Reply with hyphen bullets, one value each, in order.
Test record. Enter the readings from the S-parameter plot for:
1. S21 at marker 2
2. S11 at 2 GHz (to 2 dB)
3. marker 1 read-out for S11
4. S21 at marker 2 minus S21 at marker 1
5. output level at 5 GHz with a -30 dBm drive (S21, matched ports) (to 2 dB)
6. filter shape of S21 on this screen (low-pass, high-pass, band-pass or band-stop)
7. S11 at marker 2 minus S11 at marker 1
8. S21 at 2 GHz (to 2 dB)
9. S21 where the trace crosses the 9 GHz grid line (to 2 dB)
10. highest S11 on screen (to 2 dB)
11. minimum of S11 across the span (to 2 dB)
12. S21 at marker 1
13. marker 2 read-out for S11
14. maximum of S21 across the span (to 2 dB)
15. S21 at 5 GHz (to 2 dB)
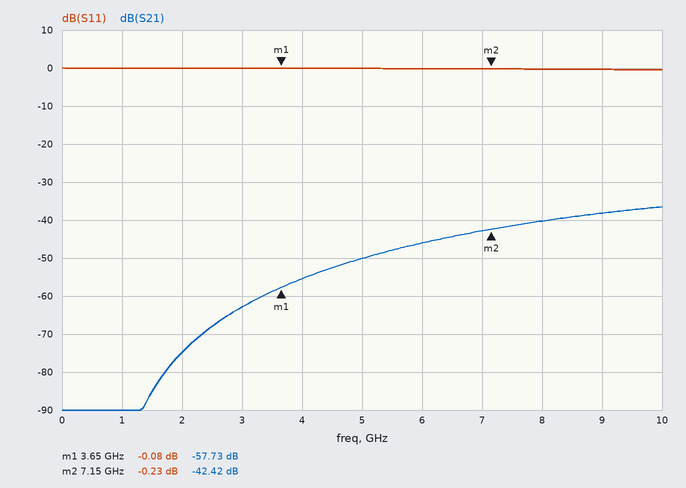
- -42.42 dB
- 0 dB
- -0.08 dB
- 15.31 dB
- -80 dBm
- high-pass
- -0.15 dB
- -74 dB
- -38 dB
- 0 dB
- 0 dB
- -57.73 dB
- -0.23 dB
- -36 dB
- -50 dB
